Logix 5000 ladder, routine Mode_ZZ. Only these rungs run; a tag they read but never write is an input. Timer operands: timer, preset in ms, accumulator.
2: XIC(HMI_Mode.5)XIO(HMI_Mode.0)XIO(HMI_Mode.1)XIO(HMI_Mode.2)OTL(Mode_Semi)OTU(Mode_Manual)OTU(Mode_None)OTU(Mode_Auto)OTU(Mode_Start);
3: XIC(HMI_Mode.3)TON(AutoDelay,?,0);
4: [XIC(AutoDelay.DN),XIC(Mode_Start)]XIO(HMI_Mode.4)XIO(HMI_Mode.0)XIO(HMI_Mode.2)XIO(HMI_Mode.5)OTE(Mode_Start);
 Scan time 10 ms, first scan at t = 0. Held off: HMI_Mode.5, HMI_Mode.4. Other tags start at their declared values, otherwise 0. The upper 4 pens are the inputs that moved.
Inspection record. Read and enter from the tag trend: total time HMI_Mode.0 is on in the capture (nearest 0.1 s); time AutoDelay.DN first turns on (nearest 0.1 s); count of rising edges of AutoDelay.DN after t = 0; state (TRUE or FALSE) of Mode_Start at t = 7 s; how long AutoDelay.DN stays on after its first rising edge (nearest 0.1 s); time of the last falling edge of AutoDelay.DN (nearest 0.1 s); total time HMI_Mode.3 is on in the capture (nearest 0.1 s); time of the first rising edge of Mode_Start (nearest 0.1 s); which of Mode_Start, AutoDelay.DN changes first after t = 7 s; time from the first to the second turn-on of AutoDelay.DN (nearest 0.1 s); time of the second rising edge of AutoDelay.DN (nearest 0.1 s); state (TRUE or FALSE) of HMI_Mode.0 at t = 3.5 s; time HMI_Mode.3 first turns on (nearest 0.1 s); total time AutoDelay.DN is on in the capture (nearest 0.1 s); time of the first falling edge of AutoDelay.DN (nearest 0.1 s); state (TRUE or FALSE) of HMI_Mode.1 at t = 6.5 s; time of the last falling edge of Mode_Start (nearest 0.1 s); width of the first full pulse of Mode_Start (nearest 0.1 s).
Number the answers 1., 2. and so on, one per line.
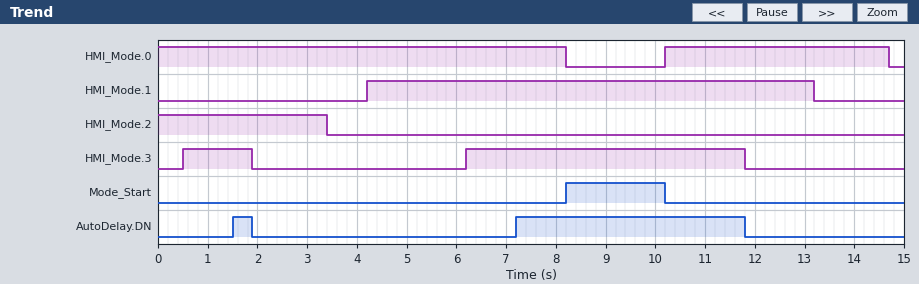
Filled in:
1. 12.7 s
2. 1.5 s
3. 2
4. FALSE
5. 0.4 s
6. 11.8 s
7. 7.0 s
8. 8.2 s
9. AutoDelay.DN
10. 5.7 s
11. 7.2 s
12. TRUE
13. 0.5 s
14. 5.0 s
15. 1.9 s
16. TRUE
17. 10.2 s
18. 2.0 s
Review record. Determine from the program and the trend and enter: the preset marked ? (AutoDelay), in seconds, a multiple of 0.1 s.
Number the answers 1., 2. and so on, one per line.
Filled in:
1. 1.0 s
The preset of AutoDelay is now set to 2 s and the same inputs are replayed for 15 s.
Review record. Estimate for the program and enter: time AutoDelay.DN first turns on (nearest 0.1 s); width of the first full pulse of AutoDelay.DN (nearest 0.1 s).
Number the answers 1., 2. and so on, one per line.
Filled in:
1. 8.2 s
2. 3.6 s
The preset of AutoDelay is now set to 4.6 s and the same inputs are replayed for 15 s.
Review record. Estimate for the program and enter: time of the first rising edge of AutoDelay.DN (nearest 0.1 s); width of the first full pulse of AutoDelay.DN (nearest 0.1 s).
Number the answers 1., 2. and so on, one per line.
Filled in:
1. 10.8 s
2. 1.0 s
